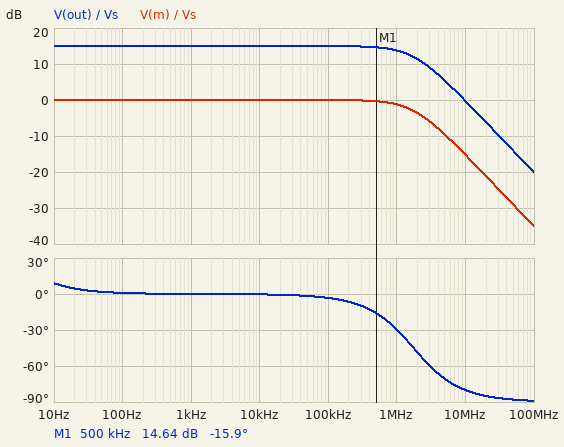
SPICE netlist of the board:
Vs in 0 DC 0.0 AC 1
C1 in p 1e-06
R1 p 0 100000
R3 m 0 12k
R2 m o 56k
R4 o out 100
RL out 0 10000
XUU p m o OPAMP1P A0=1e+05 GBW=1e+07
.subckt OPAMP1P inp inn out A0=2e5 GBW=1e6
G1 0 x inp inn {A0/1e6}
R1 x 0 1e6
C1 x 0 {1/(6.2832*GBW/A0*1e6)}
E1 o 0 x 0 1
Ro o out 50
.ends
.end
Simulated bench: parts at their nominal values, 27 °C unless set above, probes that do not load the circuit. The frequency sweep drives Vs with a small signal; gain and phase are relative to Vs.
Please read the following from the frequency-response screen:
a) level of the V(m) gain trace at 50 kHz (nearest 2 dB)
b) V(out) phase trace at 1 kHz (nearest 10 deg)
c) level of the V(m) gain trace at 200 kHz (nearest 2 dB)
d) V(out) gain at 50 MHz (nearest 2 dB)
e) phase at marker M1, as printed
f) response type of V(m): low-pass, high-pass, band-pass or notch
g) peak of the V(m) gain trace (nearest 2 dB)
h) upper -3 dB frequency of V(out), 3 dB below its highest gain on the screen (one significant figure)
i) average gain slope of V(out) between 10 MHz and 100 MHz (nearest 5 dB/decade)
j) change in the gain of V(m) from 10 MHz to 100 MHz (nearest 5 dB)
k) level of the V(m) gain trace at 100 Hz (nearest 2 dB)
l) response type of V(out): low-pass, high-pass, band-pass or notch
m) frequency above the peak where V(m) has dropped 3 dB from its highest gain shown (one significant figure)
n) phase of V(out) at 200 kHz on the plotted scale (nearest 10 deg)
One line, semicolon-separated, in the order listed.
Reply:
0 dB; 0 deg; 0 dB; -14 dB; -15.9 deg; low-pass; 0 dB; 2 MHz; -20 dB/decade; -20 dB; 0 dB; low-pass; 2 MHz; -10 deg
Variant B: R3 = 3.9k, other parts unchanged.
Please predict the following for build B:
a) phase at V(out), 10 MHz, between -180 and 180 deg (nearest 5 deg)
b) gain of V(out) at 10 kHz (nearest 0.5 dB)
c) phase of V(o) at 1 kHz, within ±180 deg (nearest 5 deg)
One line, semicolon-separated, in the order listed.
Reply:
-85 deg; 23.5 dB; 0 deg
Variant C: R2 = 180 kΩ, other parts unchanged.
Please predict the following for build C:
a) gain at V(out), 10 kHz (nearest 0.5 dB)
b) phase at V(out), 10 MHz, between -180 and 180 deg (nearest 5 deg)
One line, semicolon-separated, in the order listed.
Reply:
24.0 dB; -85 deg
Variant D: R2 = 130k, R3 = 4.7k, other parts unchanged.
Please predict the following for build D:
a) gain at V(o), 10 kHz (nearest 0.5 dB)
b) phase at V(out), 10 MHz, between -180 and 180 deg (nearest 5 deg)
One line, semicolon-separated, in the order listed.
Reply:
29.0 dB; -90 deg
